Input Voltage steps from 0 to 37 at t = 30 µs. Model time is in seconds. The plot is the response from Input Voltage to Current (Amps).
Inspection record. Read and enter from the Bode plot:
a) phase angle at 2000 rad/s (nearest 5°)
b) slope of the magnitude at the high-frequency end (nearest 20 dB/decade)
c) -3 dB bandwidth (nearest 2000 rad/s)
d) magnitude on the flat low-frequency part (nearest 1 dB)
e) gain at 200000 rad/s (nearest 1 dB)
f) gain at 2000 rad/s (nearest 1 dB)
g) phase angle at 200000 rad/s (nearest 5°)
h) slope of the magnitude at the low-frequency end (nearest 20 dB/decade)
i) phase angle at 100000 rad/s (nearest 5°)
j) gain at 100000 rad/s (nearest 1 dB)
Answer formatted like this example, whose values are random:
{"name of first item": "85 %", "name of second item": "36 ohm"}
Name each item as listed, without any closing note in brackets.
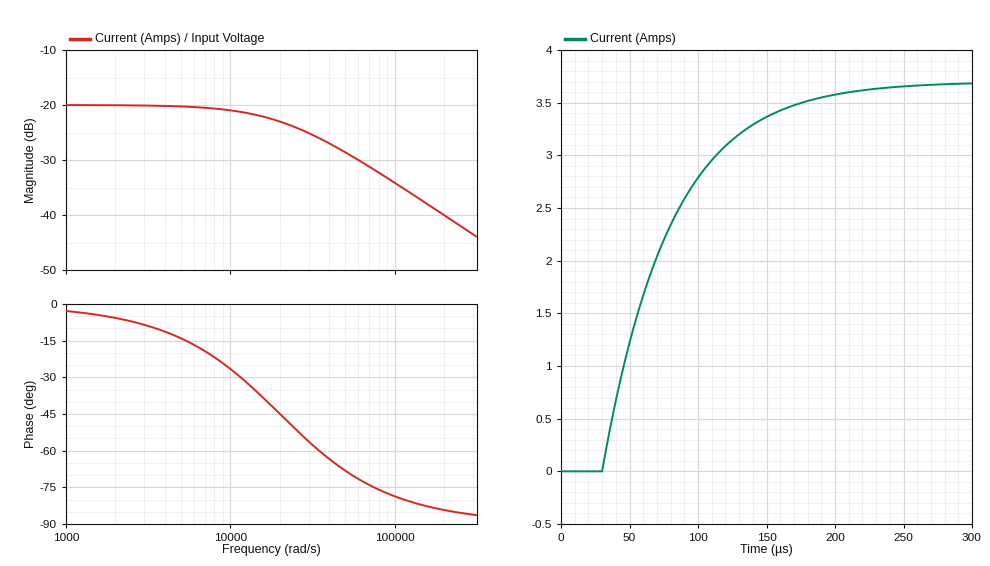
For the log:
{"phase angle at 2000 rad/s": "-5°", "slope of the magnitude at the high-frequency end": "-20 dB/decade", "-3 dB bandwidth": "20000 rad/s", "magnitude on the flat low-frequency part": "-20 dB", "gain at 200000 rad/s": "-40 dB", "gain at 2000 rad/s": "-20 dB", "phase angle at 200000 rad/s": "-85°", "slope of the magnitude at the low-frequency end": "0 dB/decade", "phase angle at 100000 rad/s": "-80°", "gain at 100000 rad/s": "-34 dB"}
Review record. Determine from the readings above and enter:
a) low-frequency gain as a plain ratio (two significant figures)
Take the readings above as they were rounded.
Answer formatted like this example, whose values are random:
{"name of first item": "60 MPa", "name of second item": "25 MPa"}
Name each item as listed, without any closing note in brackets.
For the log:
{"low-frequency gain as a plain ratio": "0.10"}
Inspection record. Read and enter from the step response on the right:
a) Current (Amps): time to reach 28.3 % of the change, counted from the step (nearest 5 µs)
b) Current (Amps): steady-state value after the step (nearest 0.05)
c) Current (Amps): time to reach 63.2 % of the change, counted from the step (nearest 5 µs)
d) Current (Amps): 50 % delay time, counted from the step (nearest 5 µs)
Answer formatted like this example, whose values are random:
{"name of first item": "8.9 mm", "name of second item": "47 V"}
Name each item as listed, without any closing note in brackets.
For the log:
{"Current (Amps): time to reach 28.3 % of the change, counted from the step": "15 µs", "Current (Amps): steady-state value after the step": "3.70", "Current (Amps): time to reach 63.2 % of the change, counted from the step": "50 µs", "Current (Amps): 50 % delay time, counted from the step": "35 µs"}
